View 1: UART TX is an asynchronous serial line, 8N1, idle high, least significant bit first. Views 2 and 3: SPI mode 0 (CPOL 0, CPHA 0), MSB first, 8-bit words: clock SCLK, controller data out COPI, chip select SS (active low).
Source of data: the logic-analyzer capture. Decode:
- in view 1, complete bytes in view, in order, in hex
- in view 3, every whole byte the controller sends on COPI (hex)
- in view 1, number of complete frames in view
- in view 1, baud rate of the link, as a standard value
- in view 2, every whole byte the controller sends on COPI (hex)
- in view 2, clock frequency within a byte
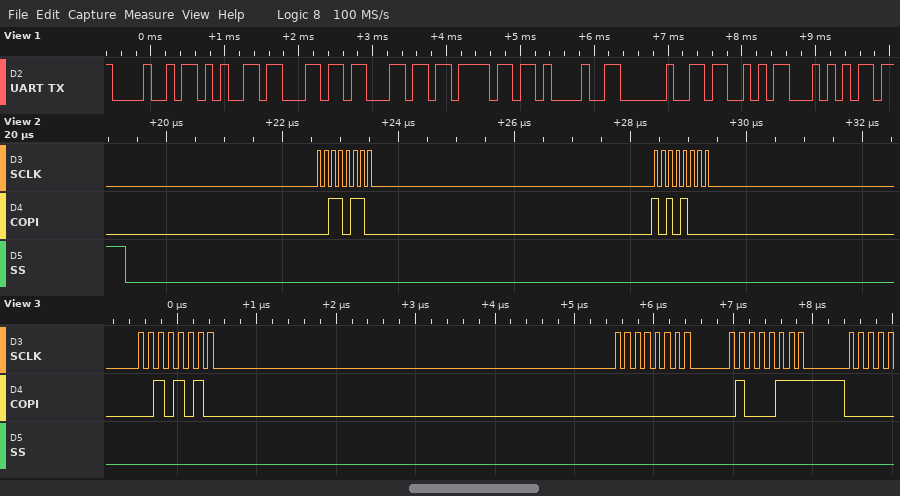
0x48 0x65 0x6C 0x6C 0x6F 0x21 0x20 0x53 0x54
0x2A 0x00 0x47
9
9600 baud
36 A8
8 MHz
